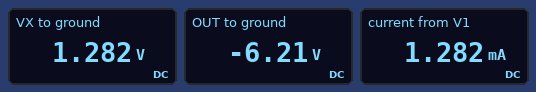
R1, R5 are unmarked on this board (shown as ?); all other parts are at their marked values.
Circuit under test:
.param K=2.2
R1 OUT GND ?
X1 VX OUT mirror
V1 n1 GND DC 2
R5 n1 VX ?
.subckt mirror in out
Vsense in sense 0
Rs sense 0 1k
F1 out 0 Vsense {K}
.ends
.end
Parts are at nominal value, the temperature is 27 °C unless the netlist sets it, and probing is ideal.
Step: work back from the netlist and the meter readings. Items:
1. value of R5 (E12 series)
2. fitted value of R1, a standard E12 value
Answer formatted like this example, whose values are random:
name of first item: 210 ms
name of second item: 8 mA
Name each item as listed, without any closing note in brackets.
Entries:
value of R5: 560 Ω
fitted value of R1, a standard E12 value: 2.2 kΩ
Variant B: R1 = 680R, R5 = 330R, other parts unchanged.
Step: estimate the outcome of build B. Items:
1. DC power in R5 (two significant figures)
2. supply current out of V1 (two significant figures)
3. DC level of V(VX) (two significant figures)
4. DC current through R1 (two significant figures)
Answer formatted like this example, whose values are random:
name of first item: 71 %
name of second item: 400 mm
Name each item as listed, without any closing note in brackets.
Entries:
DC power in R5: 750 µW
supply current out of V1: 1.5 mA
DC level of V(VX): 1.5 V
DC current through R1: 3.3 mA
